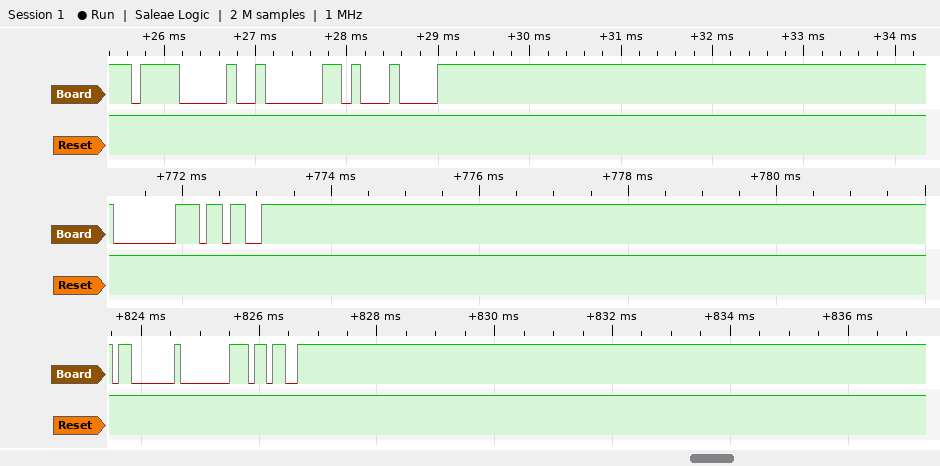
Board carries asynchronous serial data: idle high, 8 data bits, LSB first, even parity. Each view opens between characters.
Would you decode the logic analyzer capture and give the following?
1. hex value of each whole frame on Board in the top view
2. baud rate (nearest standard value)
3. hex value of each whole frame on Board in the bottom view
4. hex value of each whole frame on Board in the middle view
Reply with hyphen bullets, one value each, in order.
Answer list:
- 0F, 02, 11
- 9600 baud
- 03, 80, 9B
- 80, 9B
